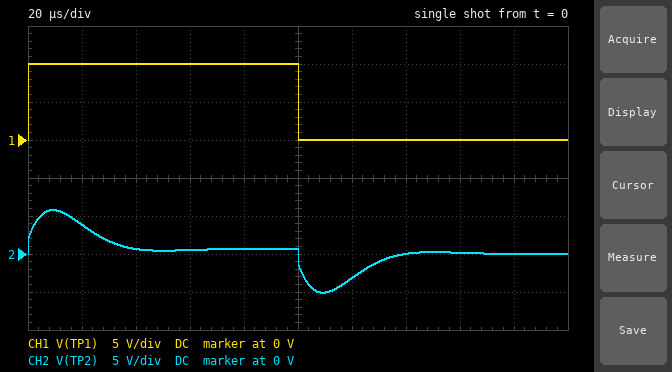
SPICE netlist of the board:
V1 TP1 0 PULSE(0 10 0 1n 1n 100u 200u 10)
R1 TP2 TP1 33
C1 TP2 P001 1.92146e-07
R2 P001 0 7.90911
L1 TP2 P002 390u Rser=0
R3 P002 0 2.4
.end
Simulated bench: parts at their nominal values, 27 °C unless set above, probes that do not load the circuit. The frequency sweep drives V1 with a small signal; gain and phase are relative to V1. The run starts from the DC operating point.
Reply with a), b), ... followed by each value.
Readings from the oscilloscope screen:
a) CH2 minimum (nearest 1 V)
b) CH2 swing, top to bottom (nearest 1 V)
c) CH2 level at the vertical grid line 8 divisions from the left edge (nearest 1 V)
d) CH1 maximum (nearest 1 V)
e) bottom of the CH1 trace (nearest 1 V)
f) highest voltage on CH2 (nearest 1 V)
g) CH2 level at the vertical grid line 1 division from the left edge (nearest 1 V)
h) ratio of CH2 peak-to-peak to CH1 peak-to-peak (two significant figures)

a) -5 V
b) 11 V
c) 0 V
d) 10 V
e) 0 V
f) 6 V
g) 4 V
h) 1.1
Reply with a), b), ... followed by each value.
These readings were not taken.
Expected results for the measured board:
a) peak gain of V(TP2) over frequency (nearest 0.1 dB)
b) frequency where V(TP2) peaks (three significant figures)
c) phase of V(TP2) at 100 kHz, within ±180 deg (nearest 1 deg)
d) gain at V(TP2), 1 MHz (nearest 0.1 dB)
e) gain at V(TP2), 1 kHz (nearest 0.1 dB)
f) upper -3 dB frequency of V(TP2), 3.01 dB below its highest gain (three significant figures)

a) -1.3 dB
b) 17.3 kHz
c) -33 deg
d) -14.2 dB
e) -20.3 dB
f) 34.1 kHz
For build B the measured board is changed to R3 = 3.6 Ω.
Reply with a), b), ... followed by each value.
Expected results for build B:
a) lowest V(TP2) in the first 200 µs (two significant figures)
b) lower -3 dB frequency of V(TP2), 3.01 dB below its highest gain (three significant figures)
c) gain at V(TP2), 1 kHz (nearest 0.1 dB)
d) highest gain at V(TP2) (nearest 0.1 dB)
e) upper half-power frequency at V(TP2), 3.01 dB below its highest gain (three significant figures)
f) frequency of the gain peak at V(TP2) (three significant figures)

a) -4.8 V
b) 9.07 kHz
c) -18.5 dB
d) -1.4 dB
e) 34.8 kHz
f) 17.6 kHz
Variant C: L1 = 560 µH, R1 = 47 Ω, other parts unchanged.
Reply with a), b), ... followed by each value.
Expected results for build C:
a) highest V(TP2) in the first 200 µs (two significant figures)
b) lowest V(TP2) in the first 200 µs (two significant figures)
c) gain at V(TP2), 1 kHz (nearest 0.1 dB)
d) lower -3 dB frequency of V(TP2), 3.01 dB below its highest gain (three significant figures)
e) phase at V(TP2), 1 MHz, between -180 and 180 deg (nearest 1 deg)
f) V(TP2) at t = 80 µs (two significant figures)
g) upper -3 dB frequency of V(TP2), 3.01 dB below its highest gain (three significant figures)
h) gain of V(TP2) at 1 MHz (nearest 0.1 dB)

a) 5.4 V
b) -4.9 V
c) -21.3 dB
d) 8.22 kHz
e) -5 deg
f) 430 mV
g) 26.4 kHz
h) -16.8 dB
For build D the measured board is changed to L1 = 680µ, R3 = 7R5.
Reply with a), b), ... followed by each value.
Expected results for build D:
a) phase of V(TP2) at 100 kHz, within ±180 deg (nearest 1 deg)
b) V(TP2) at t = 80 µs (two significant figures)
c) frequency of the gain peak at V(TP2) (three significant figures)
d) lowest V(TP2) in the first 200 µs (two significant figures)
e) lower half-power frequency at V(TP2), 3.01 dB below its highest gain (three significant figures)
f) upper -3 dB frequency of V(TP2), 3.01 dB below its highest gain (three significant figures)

a) -34 deg
b) 1.8 V
c) 13.9 kHz
d) -4.8 V
e) 6.23 kHz
f) 31.0 kHz
